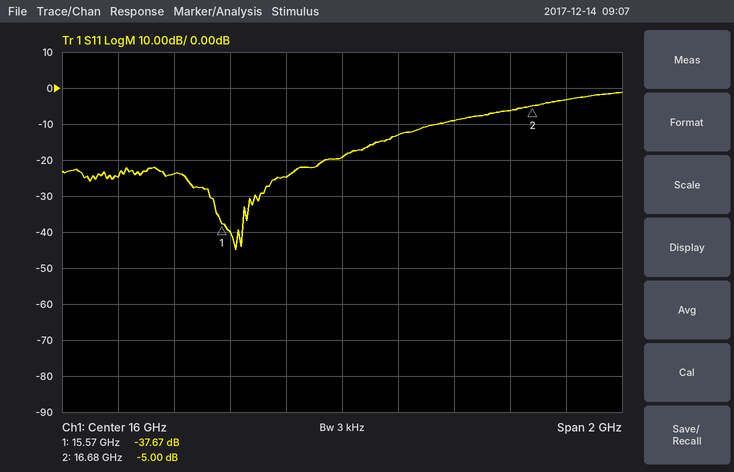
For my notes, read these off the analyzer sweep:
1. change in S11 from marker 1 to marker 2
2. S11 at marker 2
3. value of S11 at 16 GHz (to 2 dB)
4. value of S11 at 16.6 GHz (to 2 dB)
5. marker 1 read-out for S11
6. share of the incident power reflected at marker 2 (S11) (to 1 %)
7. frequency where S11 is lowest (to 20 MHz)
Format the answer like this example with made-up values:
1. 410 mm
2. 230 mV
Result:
1. 32.67 dB
2. -5.00 dB
3. -20 dB
4. -6 dB
5. -37.67 dB
6. 32 %
7. 15.62 GHz
